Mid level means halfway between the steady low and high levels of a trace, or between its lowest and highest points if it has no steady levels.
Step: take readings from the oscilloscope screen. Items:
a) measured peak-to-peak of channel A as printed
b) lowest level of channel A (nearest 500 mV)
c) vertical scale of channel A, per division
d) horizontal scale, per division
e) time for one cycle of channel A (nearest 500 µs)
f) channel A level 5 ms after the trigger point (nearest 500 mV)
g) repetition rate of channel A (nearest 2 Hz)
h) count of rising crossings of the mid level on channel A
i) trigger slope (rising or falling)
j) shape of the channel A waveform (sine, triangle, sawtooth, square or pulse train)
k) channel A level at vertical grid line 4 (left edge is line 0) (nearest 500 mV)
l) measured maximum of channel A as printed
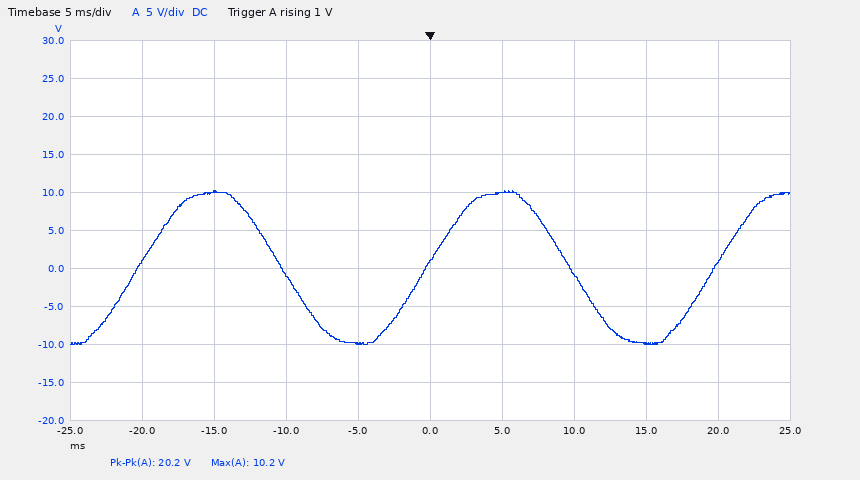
20.2 V
-10.0 V
5 V
5 ms
20.0 ms
10.0 V
50 Hz
3
rising
sine
-10.0 V
10.2 V
